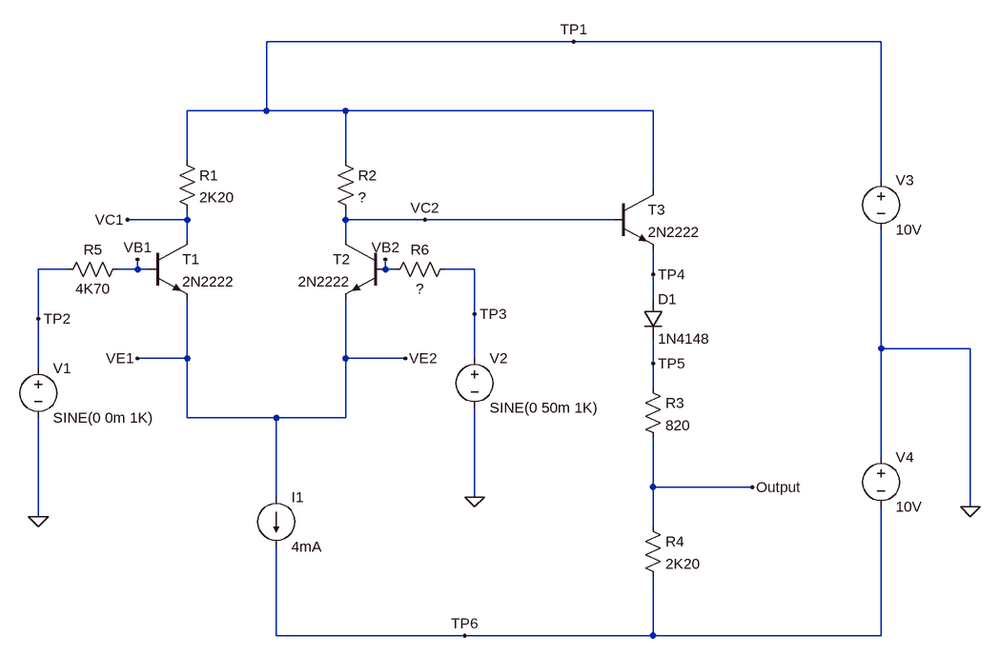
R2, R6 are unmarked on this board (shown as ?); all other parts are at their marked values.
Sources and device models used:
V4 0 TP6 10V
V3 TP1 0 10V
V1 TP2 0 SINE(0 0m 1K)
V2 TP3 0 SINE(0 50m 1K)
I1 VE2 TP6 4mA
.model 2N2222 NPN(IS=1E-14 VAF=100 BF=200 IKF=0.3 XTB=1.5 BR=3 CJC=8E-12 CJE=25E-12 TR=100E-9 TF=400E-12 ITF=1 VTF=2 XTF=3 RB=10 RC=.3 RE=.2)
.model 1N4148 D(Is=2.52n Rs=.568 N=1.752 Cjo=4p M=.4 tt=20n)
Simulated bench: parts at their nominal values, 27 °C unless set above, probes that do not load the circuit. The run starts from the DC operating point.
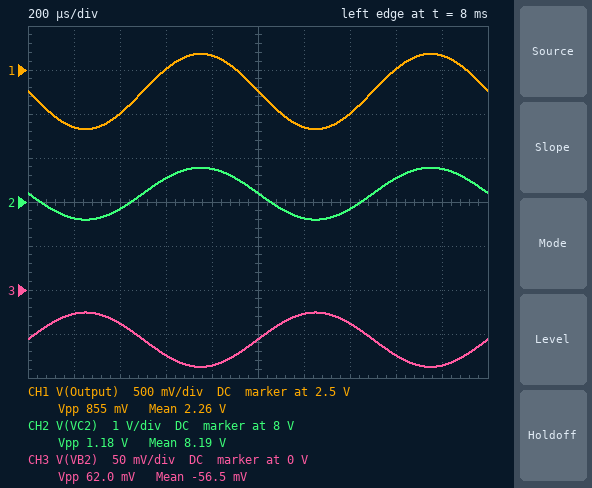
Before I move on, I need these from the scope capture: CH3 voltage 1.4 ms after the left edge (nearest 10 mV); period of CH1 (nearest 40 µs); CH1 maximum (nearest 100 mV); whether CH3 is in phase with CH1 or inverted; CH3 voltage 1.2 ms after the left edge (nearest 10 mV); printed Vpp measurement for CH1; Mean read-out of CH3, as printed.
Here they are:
-40 mV
1.00 ms
2.7 V
inverted
-30 mV
855 mV
-56.5 mV
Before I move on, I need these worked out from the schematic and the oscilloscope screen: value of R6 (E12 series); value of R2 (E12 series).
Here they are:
6.8 kΩ
1 kΩ
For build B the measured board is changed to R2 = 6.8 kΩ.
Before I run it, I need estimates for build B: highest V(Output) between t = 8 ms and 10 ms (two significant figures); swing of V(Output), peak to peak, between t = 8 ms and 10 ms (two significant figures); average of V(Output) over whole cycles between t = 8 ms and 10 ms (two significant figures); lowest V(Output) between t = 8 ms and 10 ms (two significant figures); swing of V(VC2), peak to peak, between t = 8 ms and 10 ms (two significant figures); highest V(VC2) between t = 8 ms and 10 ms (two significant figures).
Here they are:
-2.2 V
2.0 V
-3.6 V
-4.1 V
2.7 V
2.1 V
